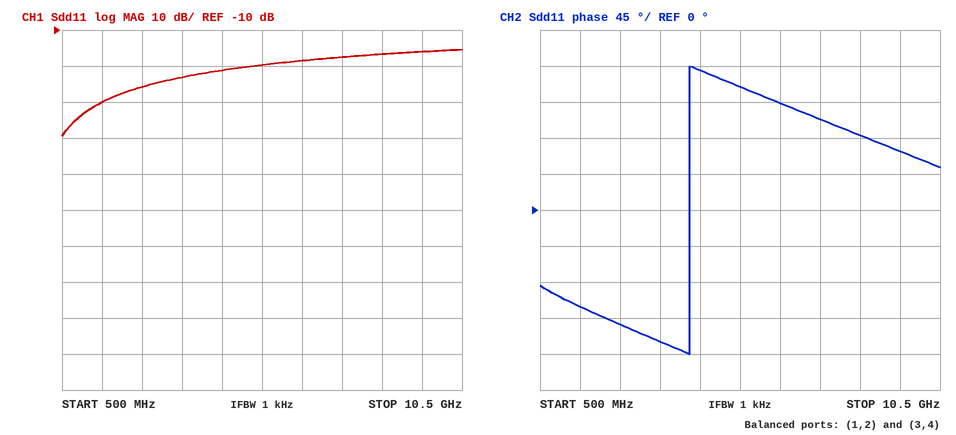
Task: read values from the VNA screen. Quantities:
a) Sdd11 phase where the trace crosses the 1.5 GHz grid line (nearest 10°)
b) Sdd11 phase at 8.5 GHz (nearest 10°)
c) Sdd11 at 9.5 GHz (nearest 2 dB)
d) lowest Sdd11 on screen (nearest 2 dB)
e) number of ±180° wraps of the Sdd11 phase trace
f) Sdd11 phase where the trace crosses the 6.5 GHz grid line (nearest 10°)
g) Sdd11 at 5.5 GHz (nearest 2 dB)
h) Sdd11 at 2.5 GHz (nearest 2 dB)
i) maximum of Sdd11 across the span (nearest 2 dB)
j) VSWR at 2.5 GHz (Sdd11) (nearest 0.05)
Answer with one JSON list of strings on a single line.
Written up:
["-120°", "90°", "-16 dB", "-40 dB", "1", "130°", "-20 dB", "-26 dB", "-16 dB", "1.10"]
